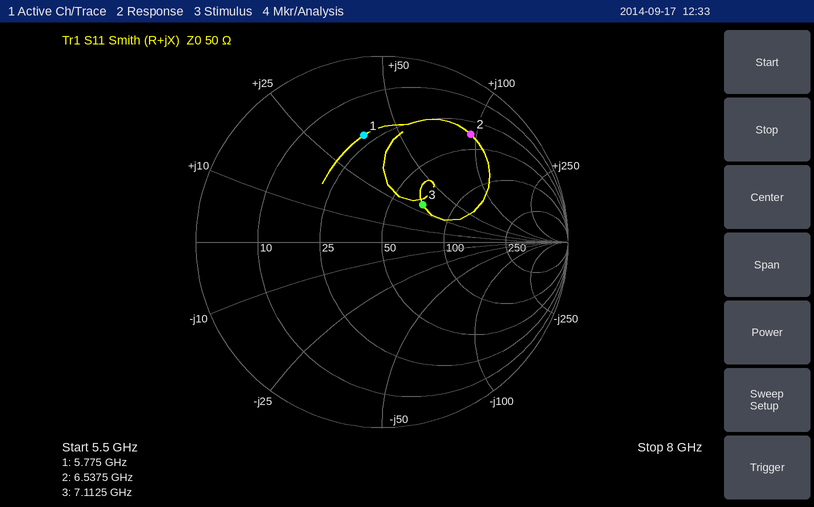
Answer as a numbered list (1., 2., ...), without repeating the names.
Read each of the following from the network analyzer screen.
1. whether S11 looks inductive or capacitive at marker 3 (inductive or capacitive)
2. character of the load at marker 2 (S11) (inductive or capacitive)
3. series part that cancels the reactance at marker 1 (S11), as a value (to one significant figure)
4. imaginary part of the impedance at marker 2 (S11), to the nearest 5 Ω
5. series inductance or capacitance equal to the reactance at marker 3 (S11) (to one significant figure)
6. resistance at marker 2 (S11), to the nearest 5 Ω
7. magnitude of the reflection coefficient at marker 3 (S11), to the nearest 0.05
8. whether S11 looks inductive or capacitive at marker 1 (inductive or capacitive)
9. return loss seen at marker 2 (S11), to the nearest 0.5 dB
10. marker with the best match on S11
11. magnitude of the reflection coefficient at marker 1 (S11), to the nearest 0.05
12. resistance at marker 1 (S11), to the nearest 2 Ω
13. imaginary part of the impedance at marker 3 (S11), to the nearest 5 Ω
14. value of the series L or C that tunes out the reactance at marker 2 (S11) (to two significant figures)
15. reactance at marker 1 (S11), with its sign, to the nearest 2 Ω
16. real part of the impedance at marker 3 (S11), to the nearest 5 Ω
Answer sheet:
1. inductive
2. inductive
3. 700 fF
4. +95 Ω
5. 700 pH
6. 35 Ω
7. 0.30
8. inductive
9. 2.5 dB
10. marker 3
11. 0.60
12. 22 Ω
13. +30 Ω
14. 260 fF
15. +38 Ω
16. 70 Ω
